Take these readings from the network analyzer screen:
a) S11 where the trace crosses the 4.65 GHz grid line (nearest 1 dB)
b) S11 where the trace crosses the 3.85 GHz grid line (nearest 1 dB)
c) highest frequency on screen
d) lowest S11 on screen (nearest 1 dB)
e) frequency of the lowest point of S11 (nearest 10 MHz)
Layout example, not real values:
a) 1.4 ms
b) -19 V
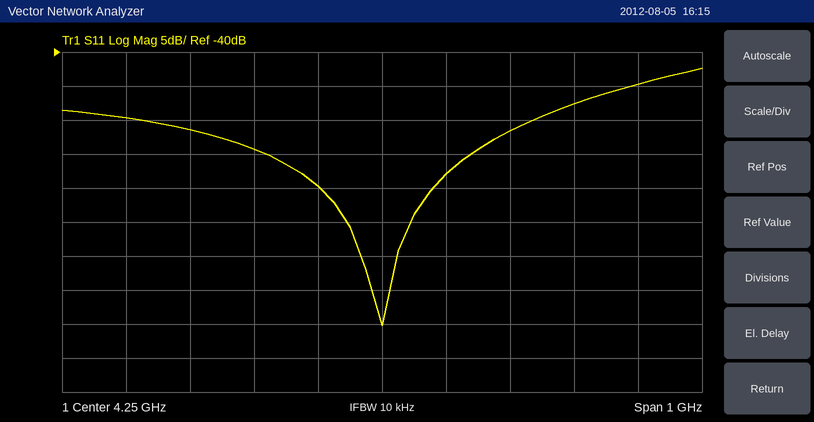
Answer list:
a) -45 dB
b) -50 dB
c) 4.75 GHz
d) -80 dB
e) 4.25 GHz
